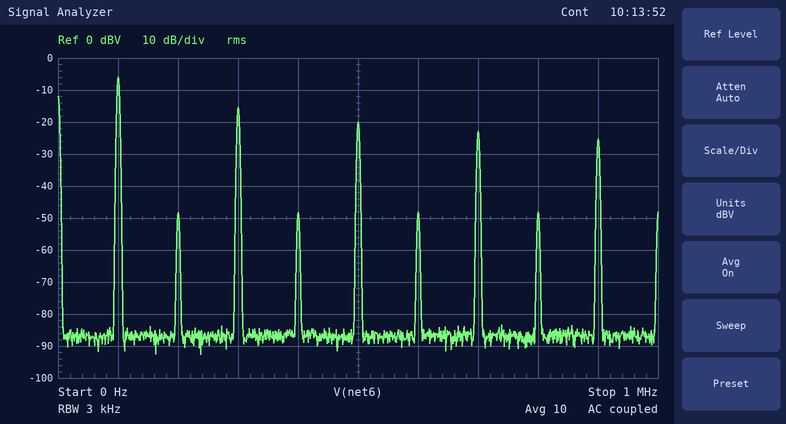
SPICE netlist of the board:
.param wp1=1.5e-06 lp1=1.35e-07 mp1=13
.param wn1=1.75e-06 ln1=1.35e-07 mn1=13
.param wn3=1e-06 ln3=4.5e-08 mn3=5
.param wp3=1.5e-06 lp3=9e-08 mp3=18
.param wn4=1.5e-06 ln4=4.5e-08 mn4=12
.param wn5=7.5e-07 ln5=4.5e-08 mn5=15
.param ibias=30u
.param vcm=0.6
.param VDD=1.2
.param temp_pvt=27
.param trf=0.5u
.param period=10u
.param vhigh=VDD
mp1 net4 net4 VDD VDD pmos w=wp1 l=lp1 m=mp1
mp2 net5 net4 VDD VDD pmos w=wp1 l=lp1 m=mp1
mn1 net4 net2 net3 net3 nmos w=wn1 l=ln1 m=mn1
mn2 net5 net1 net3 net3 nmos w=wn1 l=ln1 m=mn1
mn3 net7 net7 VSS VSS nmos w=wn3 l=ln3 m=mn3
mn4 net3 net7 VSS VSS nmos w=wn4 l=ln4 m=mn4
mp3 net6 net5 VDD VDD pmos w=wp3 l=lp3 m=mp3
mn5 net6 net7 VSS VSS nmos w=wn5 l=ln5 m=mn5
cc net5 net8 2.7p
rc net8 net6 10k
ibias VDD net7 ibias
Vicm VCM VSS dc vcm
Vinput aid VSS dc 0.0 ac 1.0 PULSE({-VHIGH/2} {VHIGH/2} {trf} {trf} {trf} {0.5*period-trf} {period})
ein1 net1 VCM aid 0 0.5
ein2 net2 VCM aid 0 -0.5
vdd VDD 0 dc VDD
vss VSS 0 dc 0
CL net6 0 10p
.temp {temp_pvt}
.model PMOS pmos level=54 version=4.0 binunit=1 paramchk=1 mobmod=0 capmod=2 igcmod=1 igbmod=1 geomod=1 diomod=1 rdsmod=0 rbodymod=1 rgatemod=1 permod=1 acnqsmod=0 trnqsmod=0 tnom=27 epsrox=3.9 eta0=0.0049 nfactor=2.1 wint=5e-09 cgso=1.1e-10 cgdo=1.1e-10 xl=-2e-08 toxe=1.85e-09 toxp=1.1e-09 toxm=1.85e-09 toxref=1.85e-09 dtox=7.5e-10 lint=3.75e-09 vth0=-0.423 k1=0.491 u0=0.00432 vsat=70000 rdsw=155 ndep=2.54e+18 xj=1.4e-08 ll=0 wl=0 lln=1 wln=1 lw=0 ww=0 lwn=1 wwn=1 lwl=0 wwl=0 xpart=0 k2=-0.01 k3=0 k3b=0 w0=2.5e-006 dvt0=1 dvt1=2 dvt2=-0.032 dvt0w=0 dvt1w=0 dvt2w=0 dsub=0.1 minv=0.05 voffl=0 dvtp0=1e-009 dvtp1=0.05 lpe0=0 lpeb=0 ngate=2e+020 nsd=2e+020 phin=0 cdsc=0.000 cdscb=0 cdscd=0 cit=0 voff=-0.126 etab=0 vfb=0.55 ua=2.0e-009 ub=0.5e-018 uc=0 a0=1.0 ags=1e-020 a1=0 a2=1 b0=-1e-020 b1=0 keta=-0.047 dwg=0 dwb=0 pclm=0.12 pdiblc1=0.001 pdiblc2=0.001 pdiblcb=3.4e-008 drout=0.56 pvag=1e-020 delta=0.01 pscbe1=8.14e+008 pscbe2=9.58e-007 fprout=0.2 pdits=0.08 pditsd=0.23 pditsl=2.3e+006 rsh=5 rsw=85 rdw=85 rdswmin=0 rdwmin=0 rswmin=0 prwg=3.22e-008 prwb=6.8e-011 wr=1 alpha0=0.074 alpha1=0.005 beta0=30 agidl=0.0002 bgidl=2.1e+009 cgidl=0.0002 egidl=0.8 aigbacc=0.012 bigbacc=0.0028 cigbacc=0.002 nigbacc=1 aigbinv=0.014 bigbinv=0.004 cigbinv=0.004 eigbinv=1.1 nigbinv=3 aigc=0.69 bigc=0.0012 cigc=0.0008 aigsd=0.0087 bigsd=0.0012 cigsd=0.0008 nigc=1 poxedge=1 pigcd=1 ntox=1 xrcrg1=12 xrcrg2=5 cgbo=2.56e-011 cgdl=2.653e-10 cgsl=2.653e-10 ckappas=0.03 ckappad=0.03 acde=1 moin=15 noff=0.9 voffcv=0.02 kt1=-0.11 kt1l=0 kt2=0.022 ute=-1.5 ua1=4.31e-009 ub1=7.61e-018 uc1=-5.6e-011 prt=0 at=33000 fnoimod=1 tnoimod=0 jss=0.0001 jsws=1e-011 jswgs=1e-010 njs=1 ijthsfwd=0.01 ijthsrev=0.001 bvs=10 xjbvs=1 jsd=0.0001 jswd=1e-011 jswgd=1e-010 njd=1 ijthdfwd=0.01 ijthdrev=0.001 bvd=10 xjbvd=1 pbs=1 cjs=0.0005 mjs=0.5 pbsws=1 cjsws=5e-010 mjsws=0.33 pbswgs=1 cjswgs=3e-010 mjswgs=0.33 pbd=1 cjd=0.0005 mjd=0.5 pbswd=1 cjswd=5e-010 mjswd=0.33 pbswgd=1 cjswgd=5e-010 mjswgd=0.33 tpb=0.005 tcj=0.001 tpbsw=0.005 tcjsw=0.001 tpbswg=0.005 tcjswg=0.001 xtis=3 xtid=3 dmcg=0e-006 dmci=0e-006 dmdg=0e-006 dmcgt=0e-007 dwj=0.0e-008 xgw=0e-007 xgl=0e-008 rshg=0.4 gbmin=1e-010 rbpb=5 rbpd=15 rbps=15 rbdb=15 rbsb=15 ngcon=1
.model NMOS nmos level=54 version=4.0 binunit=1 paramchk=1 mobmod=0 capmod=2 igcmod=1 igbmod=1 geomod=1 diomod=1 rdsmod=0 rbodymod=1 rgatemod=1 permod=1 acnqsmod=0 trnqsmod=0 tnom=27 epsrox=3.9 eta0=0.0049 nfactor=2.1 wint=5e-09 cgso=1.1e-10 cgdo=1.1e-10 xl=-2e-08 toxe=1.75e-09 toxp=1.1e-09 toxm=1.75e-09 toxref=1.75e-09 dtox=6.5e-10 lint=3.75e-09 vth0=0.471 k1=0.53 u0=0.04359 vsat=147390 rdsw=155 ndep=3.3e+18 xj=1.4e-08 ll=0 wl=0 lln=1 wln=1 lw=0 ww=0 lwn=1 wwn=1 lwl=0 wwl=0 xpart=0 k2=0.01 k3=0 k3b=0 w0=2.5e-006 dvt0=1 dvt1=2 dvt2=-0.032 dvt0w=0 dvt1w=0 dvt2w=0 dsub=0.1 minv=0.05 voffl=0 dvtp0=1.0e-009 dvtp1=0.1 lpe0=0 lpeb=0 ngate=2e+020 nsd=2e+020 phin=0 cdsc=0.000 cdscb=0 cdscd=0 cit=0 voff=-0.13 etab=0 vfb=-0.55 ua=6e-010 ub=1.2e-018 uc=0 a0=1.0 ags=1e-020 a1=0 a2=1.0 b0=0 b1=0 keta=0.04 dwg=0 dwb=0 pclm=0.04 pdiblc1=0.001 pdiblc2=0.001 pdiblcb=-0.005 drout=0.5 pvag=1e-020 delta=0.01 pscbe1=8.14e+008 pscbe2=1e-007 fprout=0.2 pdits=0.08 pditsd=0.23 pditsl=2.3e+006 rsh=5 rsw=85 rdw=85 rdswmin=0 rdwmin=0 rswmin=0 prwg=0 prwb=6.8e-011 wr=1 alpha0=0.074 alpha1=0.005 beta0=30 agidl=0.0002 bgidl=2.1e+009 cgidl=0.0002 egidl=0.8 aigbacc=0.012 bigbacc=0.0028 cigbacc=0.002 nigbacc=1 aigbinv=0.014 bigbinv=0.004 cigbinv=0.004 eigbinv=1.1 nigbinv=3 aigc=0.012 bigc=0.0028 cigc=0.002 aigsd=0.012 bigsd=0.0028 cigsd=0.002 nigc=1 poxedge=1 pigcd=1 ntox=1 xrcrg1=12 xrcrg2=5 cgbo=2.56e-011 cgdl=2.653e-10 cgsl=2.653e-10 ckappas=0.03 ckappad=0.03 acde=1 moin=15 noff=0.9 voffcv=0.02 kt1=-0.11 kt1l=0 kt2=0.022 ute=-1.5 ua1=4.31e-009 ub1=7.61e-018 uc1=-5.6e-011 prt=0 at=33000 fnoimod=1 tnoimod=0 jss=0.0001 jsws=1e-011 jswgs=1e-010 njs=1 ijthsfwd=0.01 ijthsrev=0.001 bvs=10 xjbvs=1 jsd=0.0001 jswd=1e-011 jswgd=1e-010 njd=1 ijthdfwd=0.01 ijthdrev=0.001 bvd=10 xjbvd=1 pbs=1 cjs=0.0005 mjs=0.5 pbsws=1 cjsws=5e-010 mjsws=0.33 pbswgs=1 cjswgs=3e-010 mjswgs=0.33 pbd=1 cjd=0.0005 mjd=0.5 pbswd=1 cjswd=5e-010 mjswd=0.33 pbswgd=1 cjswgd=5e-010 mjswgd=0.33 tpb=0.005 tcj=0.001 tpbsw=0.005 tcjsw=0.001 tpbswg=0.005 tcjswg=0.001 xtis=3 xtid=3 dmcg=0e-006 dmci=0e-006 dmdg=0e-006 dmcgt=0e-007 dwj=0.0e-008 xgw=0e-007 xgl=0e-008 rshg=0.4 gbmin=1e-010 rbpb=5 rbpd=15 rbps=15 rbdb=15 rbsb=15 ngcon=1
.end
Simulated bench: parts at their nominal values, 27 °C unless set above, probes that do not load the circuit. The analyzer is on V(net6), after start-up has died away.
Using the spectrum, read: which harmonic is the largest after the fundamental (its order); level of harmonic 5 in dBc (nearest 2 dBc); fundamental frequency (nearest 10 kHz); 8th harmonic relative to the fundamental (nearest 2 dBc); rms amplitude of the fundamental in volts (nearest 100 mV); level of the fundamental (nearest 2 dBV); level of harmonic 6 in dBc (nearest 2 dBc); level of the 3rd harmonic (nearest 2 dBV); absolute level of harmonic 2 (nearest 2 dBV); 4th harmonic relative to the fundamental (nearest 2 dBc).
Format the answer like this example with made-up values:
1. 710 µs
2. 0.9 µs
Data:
1. 3
2. -14 dBc
3. 100 kHz
4. -42 dBc
5. 500 mV
6. -6 dBV
7. -42 dBc
8. -16 dBV
9. -48 dBV
10. -42 dBc
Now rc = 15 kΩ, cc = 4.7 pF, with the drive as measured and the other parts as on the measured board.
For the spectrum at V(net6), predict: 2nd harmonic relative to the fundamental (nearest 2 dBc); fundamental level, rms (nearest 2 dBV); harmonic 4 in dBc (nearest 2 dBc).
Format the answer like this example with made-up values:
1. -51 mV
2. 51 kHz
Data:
1. -38 dBc
2. -6 dBV
3. -38 dBc
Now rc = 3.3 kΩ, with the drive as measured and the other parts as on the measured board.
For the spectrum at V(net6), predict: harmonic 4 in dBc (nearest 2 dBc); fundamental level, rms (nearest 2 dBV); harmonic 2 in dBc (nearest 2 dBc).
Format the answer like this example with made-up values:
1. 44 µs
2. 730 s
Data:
1. -44 dBc
2. -6 dBV
3. -44 dBc
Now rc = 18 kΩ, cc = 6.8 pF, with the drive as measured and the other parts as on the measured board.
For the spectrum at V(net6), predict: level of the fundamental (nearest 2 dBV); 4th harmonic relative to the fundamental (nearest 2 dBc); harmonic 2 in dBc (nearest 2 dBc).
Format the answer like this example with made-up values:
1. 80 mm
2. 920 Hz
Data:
1. -6 dBV
2. -36 dBc
3. -36 dBc
